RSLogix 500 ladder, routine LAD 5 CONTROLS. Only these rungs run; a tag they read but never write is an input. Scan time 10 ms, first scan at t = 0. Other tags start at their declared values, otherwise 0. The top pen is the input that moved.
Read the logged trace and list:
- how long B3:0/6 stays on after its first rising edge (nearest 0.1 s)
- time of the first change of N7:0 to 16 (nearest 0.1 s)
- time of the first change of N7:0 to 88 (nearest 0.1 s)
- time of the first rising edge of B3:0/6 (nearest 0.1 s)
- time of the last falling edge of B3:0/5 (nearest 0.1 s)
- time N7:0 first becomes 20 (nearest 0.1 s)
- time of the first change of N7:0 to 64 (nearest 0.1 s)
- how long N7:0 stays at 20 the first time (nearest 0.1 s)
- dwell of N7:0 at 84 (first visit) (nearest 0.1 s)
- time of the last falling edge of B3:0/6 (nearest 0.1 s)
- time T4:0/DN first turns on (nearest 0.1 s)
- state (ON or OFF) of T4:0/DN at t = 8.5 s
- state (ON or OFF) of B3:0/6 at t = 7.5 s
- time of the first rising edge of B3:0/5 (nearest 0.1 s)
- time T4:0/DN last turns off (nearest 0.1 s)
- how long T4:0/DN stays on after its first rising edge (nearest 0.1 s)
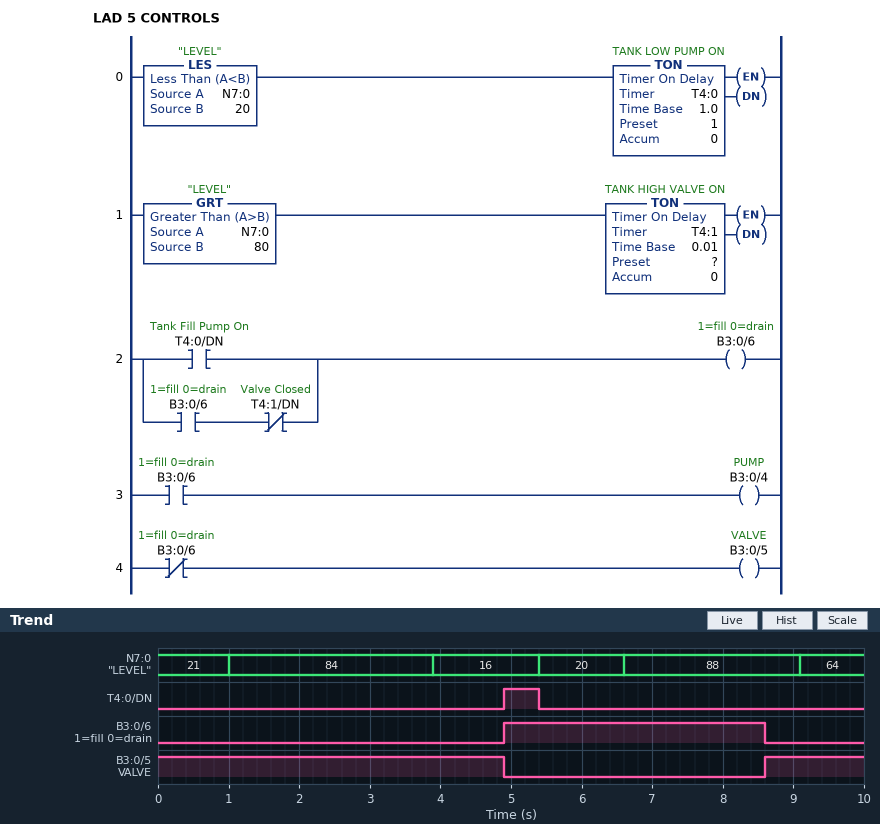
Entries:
3.7 s
3.9 s
6.6 s
4.9 s
4.9 s
5.4 s
9.1 s
1.2 s
2.9 s
8.6 s
4.9 s
OFF
ON
8.6 s
5.4 s
0.5 s
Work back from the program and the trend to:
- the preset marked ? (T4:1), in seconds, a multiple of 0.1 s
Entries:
2.0 s
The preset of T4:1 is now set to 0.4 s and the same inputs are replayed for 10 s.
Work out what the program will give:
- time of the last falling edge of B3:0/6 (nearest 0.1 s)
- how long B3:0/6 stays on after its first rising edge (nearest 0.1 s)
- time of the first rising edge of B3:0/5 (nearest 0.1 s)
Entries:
7.0 s
2.1 s
7.0 s
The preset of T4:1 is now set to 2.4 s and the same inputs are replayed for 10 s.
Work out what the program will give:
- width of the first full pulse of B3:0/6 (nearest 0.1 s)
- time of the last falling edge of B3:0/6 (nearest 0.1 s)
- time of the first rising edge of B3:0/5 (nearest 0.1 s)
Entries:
4.1 s
9.0 s
9.0 s
